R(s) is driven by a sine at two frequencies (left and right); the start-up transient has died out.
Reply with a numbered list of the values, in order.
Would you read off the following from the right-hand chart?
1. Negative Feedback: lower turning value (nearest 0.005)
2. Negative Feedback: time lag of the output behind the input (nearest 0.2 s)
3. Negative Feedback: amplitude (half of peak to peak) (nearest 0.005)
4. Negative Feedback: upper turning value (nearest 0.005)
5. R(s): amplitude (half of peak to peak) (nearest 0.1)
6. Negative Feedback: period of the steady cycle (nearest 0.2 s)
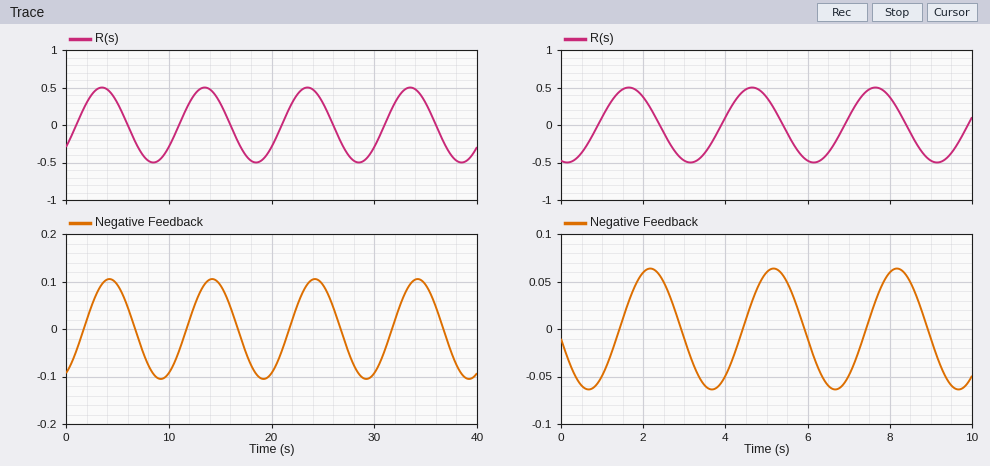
1. -0.065
2. 0.6 s
3. 0.065
4. 0.065
5. 0.5
6. 3.0 s
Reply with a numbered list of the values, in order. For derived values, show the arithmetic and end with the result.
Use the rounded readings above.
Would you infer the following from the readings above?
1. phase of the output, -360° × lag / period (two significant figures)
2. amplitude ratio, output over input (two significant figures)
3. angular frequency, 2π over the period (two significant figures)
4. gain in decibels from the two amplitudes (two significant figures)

1. -360 × 0.6 / 3 = -72°
2. 0.065 / 0.5 = 0.13
3. 2π / 3 = 2.1 rad/s
4. 20 log10(0.065 / 0.5) = -18 dB
